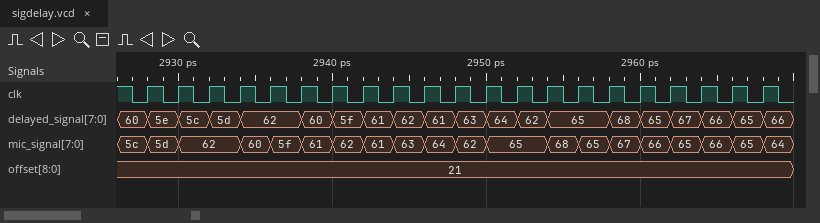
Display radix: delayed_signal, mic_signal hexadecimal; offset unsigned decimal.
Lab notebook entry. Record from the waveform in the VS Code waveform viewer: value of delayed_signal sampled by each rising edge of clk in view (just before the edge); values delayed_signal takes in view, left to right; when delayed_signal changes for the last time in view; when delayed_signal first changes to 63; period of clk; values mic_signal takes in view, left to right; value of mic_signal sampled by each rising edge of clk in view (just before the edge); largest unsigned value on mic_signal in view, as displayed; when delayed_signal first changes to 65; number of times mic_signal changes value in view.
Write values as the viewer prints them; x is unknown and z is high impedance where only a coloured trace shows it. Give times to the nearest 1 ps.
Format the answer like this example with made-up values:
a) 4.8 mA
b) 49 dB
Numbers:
a) 60, 5e, 5c, 5d, 62, 62, 60, 5f, 61, 62, 61, 63, 64, 62, 65, 65, 68, 65, 67, 66, 65
b) 60, 5e, 5c, 5d, 62, 60, 5f, 61, 62, 61, 63, 64, 62, 65, 68, 65, 67, 66, 65, 66
c) 2968 ps
d) 2948 ps
e) 2 ps
f) 5c, 5d, 62, 60, 5f, 61, 62, 61, 63, 64, 62, 65, 68, 65, 67, 66, 65, 66, 65, 64
g) 5c, 5d, 62, 62, 60, 5f, 61, 62, 61, 63, 64, 62, 65, 65, 68, 65, 67, 66, 65, 66, 65
h) 68
i) 2954 ps
j) 19
